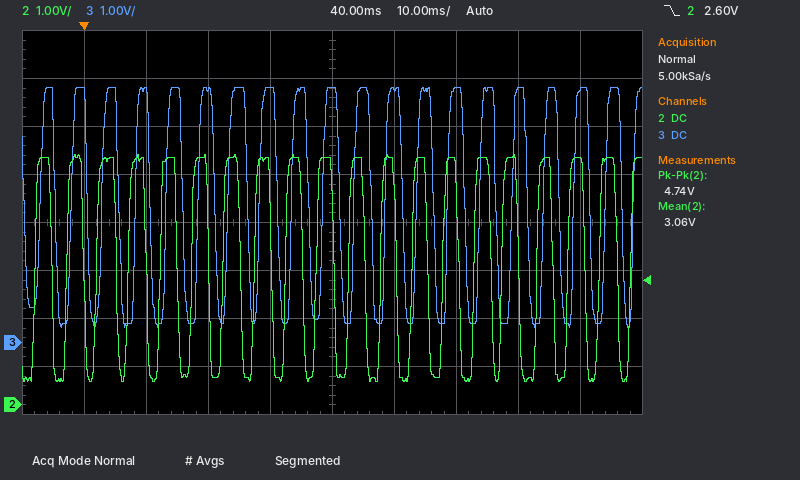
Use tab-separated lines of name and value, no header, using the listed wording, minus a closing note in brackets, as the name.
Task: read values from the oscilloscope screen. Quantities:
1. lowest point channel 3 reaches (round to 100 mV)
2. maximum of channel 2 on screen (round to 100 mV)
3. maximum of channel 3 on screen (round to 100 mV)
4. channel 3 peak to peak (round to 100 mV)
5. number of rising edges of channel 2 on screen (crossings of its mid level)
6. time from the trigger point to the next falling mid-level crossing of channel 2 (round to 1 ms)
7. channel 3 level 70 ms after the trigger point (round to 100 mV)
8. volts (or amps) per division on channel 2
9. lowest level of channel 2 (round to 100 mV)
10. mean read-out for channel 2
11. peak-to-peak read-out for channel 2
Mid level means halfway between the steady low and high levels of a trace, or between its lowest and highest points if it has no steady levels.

lowest point channel 3 reaches	300 mV
maximum of channel 2 on screen	5.2 V
maximum of channel 3 on screen	5.3 V
channel 3 peak to peak	5.0 V
number of rising edges of channel 2 on screen	20
time from the trigger point to the next falling mid-level crossing of channel 2	5 ms
channel 3 level 70 ms after the trigger point	5.2 V
volts (or amps) per division on channel 2	1 V
lowest level of channel 2	500 mV
mean read-out for channel 2	3.06 V
peak-to-peak read-out for channel 2	4.74 V
